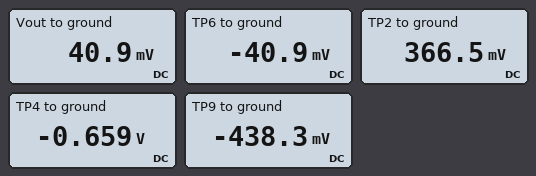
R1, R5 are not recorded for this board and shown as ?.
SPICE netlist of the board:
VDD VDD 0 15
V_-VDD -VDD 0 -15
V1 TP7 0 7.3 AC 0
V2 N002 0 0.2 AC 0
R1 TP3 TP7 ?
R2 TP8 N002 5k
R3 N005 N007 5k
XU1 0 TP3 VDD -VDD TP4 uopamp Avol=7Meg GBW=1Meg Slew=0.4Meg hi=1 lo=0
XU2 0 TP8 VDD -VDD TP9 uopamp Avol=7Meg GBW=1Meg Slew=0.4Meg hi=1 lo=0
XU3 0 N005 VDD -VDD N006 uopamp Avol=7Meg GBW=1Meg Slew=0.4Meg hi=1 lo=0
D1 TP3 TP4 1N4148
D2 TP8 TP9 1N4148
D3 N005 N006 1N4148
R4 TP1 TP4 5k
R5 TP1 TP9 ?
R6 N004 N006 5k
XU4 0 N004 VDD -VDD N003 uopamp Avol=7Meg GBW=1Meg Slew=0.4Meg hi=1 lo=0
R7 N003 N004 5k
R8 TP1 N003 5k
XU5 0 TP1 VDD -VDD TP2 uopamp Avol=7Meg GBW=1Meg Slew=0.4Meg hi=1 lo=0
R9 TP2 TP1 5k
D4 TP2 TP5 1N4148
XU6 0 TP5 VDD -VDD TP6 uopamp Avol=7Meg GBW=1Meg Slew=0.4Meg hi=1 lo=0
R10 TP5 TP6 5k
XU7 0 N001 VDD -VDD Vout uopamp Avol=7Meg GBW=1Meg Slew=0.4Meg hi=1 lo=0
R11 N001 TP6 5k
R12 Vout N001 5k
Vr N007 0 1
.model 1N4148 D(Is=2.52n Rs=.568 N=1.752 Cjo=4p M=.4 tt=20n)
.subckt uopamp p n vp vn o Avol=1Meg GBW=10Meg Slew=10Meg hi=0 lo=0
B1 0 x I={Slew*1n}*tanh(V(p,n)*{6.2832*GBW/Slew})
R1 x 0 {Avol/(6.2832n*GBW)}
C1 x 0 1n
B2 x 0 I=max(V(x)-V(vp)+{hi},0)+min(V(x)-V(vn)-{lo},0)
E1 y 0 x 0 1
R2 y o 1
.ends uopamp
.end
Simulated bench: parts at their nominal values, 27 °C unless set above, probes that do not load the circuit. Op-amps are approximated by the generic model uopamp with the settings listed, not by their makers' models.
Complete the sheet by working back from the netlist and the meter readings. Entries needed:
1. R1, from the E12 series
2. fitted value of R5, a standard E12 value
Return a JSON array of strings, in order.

["1.5 kΩ", "10 kΩ"]
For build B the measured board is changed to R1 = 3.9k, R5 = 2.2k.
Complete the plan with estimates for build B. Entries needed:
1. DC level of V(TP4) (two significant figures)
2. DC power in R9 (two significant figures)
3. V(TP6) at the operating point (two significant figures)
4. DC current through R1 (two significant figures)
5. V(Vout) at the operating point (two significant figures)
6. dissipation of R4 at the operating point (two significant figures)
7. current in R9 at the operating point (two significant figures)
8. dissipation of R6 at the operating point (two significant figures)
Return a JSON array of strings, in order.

["-610 mV", "240 µW", "-15 V", "1.9 mA", "14 V", "75 µW", "220 µA", "52 µW"]
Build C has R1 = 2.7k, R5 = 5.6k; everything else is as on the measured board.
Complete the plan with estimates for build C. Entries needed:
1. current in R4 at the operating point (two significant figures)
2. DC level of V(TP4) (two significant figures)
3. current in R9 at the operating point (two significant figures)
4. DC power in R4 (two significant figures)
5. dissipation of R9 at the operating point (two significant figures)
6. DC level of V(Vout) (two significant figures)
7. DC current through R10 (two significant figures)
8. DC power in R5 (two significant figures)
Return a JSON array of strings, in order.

["130 µA", "-630 mV", "100 µA", "80 µW", "52 µW", "990 mV", "200 µA", "34 µW"]
